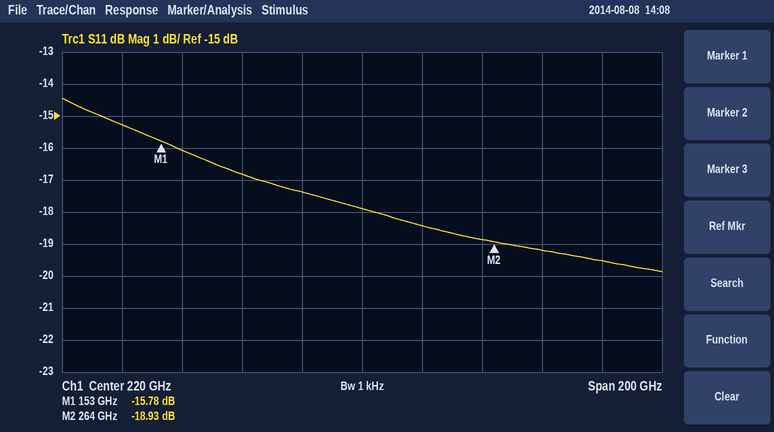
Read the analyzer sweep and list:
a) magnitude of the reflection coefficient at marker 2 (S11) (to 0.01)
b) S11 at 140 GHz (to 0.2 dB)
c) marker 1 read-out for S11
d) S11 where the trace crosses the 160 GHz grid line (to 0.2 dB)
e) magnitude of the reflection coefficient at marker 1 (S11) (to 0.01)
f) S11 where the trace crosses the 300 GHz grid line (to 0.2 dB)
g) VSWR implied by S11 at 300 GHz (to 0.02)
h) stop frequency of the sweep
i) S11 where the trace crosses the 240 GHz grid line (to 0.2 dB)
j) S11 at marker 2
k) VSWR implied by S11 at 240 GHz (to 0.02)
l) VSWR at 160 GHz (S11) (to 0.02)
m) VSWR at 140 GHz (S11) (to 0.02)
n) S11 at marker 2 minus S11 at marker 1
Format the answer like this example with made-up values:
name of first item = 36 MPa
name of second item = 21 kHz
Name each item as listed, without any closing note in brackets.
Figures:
magnitude of the reflection coefficient at marker 2 (S11) = 0.11
S11 at 140 GHz = -15.2 dB
marker 1 read-out for S11 = -15.78 dB
S11 where the trace crosses the 160 GHz grid line = -16.0 dB
magnitude of the reflection coefficient at marker 1 (S11) = 0.16
S11 where the trace crosses the 300 GHz grid line = -19.6 dB
VSWR implied by S11 at 300 GHz = 1.24
stop frequency of the sweep = 320 GHz
S11 where the trace crosses the 240 GHz grid line = -18.4 dB
S11 at marker 2 = -18.93 dB
VSWR implied by S11 at 240 GHz = 1.28
VSWR at 160 GHz (S11) = 1.38
VSWR at 140 GHz (S11) = 1.42
S11 at marker 2 minus S11 at marker 1 = -3.15 dB
